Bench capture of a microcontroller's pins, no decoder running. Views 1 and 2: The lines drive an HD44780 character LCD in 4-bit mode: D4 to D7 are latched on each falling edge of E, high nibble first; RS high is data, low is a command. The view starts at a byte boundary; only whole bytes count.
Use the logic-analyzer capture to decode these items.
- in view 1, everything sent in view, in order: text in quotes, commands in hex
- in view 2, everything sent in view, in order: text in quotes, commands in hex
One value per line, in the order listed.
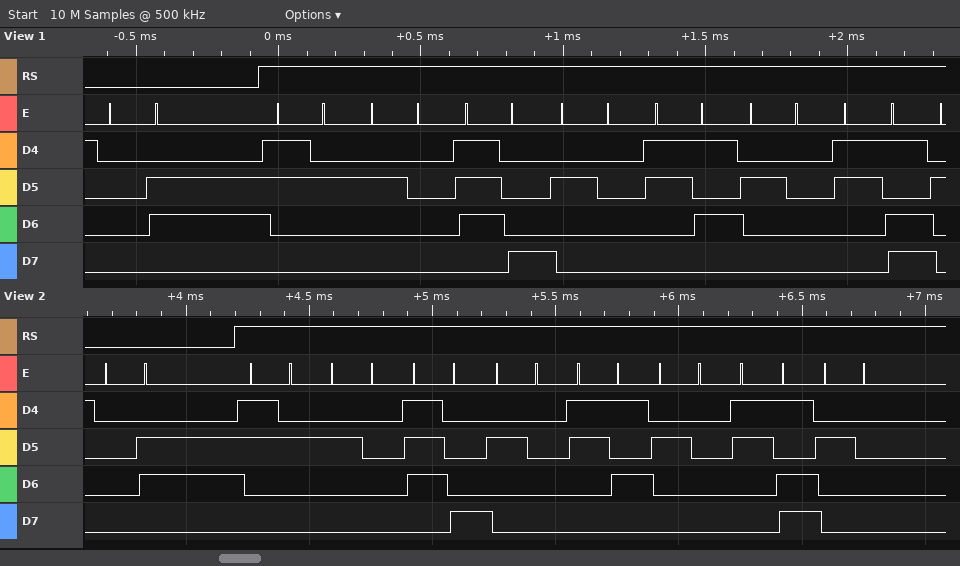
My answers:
0x06 "2 x 5 ="
0x06 "2 x 5 = "
